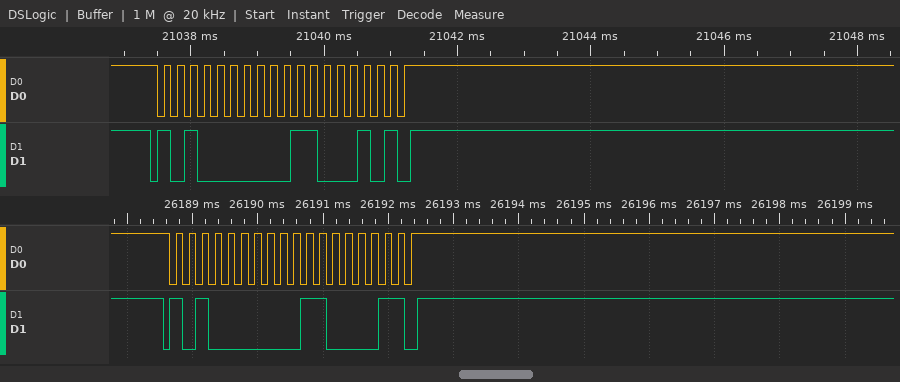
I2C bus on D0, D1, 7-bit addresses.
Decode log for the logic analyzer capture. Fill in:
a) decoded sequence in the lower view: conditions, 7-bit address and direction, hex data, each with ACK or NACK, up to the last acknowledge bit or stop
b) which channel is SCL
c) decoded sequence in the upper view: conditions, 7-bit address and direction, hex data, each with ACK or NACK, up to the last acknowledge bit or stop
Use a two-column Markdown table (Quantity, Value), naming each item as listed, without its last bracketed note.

| Quantity | Value |
|---|---|
| decoded sequence in the lower view: conditions, 7-bit address and direction, hex data, each with ACK or NACK, up to the last acknowledge bit or stop | start, address 50 write ACK, 61 NACK, stop |
| which channel is SCL | D0 |
| decoded sequence in the upper view: conditions, 7-bit address and direction, hex data, each with ACK or NACK, up to the last acknowledge bit or stop | start, address 50 write ACK, 62 NACK, stop |
